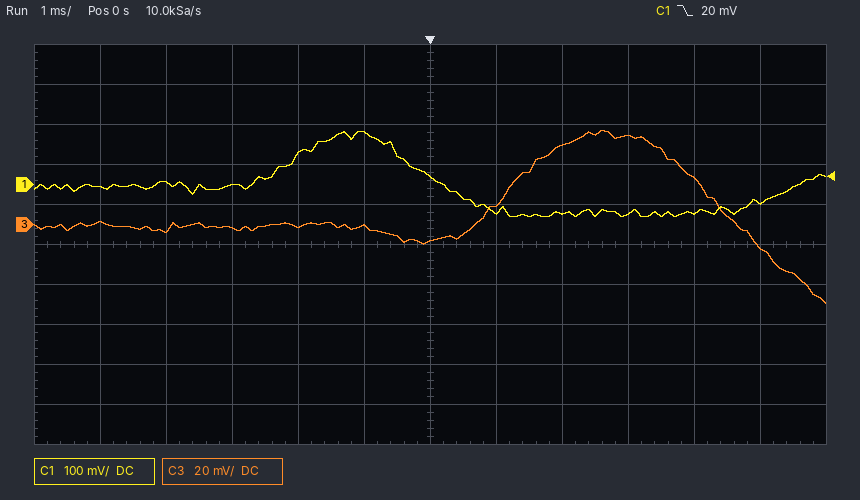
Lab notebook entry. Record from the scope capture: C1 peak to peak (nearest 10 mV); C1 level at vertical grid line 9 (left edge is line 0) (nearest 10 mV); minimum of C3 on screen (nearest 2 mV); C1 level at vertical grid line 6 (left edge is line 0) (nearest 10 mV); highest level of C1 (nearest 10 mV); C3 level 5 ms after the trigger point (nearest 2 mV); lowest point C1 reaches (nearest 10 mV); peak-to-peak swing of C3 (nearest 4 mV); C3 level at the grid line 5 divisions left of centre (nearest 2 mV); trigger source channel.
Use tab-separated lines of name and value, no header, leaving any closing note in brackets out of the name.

C1 peak to peak	210 mV
C1 level at vertical grid line 9 (left edge is line 0)	-70 mV
minimum of C3 on screen	-40 mV
C1 level at vertical grid line 6 (left edge is line 0)	20 mV
highest level of C1	130 mV
C3 level 5 ms after the trigger point	-12 mV
lowest point C1 reaches	-80 mV
peak-to-peak swing of C3	88 mV
C3 level at the grid line 5 divisions left of centre	2 mV
trigger source channel	C1
